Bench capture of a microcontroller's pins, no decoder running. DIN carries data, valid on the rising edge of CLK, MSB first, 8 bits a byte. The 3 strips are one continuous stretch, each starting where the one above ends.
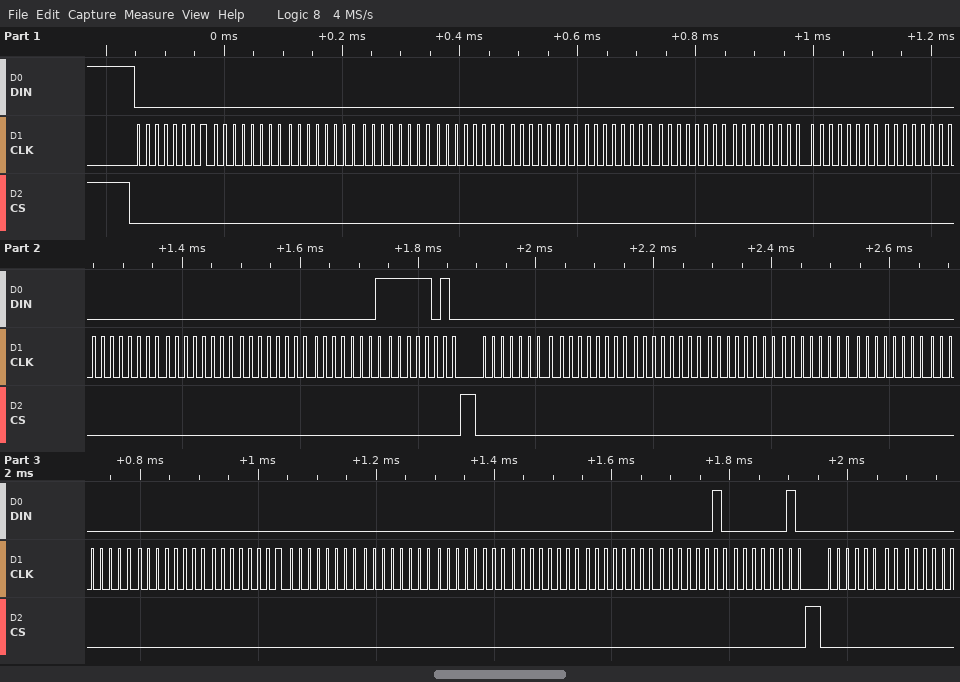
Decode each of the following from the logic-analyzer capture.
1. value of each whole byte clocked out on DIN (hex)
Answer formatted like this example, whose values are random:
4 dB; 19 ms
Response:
00 00 00 00 00 00 00 00 00 00 00 00 00 00 01 FA 00 00 00 00 00 00 00 00 00 00 00 00 00 00 02 02 00
